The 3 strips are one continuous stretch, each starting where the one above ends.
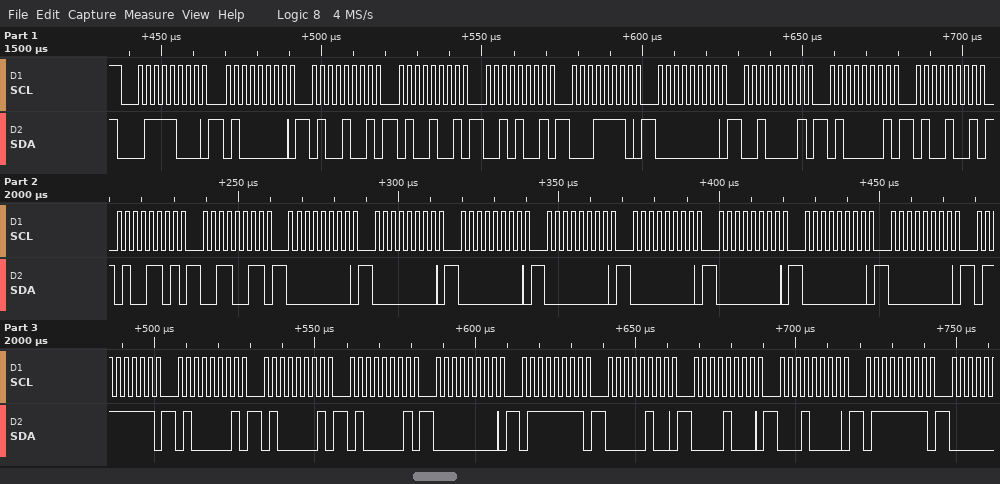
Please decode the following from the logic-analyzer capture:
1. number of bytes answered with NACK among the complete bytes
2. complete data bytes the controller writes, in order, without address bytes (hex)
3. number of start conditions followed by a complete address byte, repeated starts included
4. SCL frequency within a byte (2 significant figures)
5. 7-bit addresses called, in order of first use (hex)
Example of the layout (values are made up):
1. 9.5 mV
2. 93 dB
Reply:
1. 0
2. 40 49 49 29 1E 00 21 41 49 4D 33 00 00 00 00 00 00 00 00 7F 41 41 41 00 7F 04 08 10 7F
3. 1
4. 400 kHz
5. 0x3C
